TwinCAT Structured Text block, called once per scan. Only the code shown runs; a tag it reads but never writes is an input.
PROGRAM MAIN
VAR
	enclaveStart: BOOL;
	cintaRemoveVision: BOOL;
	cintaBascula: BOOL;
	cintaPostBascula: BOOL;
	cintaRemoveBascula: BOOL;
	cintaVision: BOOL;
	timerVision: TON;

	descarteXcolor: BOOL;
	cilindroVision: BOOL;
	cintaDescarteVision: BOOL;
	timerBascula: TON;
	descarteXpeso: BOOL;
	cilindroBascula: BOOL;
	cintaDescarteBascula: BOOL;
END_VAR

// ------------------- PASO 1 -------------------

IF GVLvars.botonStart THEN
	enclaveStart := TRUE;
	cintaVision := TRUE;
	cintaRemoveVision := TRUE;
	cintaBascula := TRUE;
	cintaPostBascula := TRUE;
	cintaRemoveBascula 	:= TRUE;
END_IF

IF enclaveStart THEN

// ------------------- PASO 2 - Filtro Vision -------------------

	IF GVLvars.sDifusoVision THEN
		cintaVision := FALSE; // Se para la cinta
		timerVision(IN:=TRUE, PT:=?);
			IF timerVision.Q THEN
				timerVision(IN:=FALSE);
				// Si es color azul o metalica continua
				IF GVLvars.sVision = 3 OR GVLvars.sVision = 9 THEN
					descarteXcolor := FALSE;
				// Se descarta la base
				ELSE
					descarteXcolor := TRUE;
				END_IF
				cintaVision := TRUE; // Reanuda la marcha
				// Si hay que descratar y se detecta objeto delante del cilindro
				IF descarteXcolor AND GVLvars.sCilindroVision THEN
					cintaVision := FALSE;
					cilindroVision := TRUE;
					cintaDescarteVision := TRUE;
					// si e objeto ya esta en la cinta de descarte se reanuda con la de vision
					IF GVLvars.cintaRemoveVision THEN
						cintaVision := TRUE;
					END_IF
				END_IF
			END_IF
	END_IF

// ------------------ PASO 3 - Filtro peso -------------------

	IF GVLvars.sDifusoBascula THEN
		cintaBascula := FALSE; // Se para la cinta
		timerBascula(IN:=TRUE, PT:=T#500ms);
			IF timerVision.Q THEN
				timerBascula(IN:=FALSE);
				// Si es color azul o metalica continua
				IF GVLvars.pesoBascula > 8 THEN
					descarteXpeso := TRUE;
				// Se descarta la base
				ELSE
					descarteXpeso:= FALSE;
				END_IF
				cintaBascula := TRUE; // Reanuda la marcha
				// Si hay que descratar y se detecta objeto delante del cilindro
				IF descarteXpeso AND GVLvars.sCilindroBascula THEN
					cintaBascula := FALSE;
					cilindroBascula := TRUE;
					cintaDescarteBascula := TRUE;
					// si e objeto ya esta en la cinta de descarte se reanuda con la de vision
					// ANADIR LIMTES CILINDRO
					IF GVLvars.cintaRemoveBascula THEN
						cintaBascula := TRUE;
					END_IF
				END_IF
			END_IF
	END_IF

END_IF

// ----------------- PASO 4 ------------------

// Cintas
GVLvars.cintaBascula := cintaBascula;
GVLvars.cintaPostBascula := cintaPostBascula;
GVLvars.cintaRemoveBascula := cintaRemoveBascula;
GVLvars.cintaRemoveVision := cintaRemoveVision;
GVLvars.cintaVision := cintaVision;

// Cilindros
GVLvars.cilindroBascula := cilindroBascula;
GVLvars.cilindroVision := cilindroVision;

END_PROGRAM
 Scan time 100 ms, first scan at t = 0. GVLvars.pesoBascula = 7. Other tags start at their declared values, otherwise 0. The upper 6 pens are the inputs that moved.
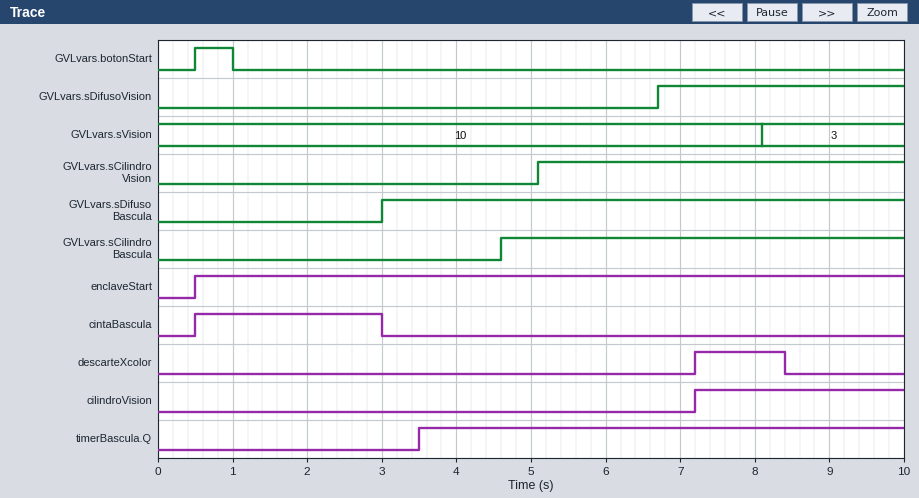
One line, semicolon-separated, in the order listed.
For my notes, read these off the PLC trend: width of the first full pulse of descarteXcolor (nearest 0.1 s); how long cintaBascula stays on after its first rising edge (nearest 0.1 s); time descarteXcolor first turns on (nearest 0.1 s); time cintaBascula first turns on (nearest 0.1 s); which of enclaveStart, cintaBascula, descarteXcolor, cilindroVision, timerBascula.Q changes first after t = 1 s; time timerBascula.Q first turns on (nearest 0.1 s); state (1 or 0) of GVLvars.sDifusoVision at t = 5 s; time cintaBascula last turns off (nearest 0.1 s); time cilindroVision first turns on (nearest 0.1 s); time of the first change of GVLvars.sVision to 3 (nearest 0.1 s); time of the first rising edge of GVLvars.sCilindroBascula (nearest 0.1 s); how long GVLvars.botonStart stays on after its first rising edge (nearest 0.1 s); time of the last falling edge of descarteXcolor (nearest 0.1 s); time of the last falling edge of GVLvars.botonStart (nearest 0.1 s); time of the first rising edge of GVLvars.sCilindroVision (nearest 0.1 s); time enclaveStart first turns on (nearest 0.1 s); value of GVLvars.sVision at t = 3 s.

1.2 s; 2.5 s; 7.2 s; 0.5 s; cintaBascula; 3.5 s; 0; 3.0 s; 7.2 s; 8.1 s; 4.6 s; 0.5 s; 8.4 s; 1.0 s; 5.1 s; 0.5 s; 10
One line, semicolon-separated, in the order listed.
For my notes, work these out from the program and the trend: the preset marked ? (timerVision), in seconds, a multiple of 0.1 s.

0.5 s
